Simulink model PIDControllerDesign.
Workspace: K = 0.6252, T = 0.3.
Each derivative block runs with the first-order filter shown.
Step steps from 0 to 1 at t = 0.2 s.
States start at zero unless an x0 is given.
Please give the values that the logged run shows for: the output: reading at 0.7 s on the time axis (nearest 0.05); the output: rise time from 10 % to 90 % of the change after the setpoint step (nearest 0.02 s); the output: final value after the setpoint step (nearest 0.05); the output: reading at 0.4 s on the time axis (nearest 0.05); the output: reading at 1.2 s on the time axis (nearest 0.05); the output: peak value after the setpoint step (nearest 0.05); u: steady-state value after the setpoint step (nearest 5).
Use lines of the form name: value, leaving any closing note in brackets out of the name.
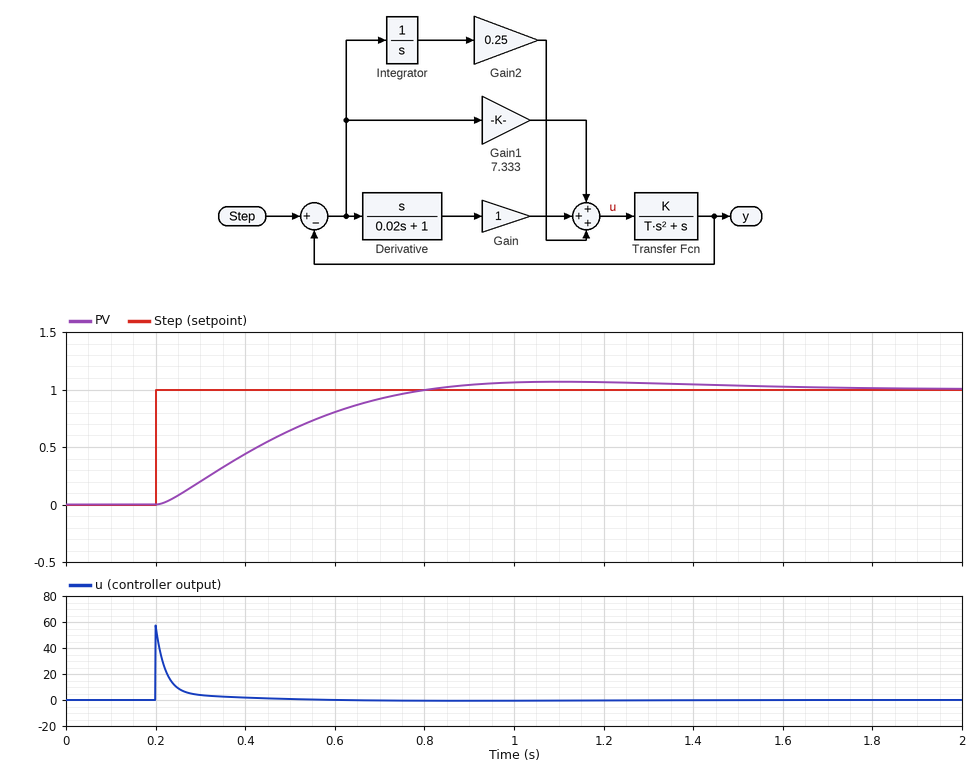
the output: reading at 0.7 s on the time axis: 0.90
the output: rise time from 10 % to 90 % of the change after the setpoint step: 0.42 s
the output: final value after the setpoint step: 1.00
the output: reading at 0.4 s on the time axis: 0.45
the output: reading at 1.2 s on the time axis: 1.05
the output: peak value after the setpoint step: 1.05
u: steady-state value after the setpoint step: 0
